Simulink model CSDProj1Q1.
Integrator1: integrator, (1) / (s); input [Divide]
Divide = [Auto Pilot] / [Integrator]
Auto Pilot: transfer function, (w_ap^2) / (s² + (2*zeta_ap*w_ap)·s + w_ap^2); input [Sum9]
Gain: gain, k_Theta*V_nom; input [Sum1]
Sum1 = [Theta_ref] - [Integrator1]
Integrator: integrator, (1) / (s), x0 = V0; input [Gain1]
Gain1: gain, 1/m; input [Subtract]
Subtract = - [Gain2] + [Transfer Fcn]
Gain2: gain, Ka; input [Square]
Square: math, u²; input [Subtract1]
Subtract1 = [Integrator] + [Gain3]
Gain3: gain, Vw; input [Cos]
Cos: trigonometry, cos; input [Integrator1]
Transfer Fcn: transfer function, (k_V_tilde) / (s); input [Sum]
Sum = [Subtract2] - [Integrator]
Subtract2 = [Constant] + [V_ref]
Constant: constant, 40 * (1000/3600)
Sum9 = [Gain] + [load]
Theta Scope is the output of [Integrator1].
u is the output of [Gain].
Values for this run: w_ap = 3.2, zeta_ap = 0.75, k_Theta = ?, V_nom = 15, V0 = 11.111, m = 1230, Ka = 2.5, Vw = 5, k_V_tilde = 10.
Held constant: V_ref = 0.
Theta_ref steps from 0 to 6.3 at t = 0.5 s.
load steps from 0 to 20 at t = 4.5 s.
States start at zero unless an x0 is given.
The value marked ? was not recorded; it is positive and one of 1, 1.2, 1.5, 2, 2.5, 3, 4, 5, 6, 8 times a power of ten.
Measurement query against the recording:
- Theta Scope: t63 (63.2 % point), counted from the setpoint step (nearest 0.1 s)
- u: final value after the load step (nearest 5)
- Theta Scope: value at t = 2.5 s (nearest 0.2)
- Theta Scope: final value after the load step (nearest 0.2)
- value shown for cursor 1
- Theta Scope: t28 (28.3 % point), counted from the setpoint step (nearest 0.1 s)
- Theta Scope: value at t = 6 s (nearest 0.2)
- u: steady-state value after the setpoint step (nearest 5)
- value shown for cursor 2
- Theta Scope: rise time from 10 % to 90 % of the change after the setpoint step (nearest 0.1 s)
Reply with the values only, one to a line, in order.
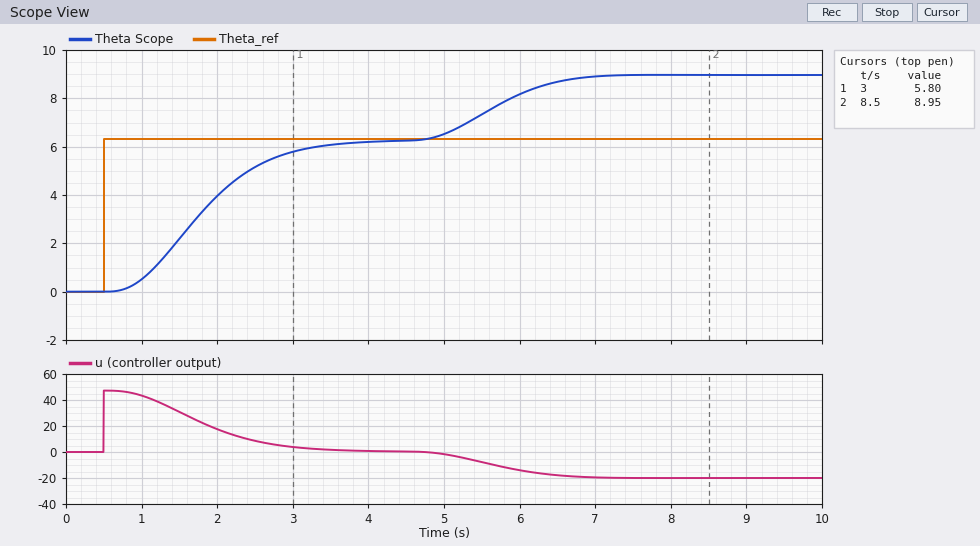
1.5 s
-20
5.2
9.0
5.80
0.9 s
8.2
0
8.95
1.8 s
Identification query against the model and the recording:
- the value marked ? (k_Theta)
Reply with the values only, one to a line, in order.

0.5
